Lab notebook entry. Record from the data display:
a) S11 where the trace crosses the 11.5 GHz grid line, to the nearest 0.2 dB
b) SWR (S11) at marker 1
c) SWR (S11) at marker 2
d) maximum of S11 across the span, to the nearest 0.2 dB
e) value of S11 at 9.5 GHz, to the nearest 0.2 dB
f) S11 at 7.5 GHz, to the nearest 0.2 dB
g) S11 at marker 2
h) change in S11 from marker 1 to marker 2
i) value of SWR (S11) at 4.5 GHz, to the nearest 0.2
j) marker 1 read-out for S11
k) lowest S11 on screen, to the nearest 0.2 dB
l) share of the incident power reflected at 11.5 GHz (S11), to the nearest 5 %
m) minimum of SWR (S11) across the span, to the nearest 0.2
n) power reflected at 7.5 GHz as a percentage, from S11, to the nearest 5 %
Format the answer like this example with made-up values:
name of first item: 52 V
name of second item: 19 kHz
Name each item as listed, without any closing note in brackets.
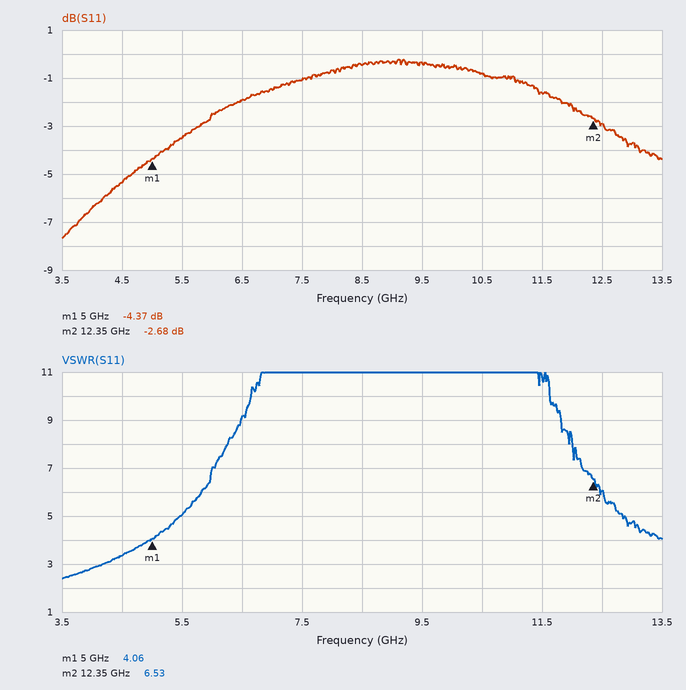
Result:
S11 where the trace crosses the 11.5 GHz grid line, to the nearest 0.2 dB: -1.6 dB
SWR (S11) at marker 1: 4.06
SWR (S11) at marker 2: 6.53
maximum of S11 across the span, to the nearest 0.2 dB: -0.2 dB
value of S11 at 9.5 GHz, to the nearest 0.2 dB: -0.4 dB
S11 at 7.5 GHz, to the nearest 0.2 dB: -1.0 dB
S11 at marker 2: -2.68 dB
change in S11 from marker 1 to marker 2: 1.69 dB
value of SWR (S11) at 4.5 GHz, to the nearest 0.2: 3.4
marker 1 read-out for S11: -4.37 dB
lowest S11 on screen, to the nearest 0.2 dB: -7.6 dB
share of the incident power reflected at 11.5 GHz (S11), to the nearest 5 %: 70 %
minimum of SWR (S11) across the span, to the nearest 0.2: 2.4
power reflected at 7.5 GHz as a percentage, from S11, to the nearest 5 %: 80 %
